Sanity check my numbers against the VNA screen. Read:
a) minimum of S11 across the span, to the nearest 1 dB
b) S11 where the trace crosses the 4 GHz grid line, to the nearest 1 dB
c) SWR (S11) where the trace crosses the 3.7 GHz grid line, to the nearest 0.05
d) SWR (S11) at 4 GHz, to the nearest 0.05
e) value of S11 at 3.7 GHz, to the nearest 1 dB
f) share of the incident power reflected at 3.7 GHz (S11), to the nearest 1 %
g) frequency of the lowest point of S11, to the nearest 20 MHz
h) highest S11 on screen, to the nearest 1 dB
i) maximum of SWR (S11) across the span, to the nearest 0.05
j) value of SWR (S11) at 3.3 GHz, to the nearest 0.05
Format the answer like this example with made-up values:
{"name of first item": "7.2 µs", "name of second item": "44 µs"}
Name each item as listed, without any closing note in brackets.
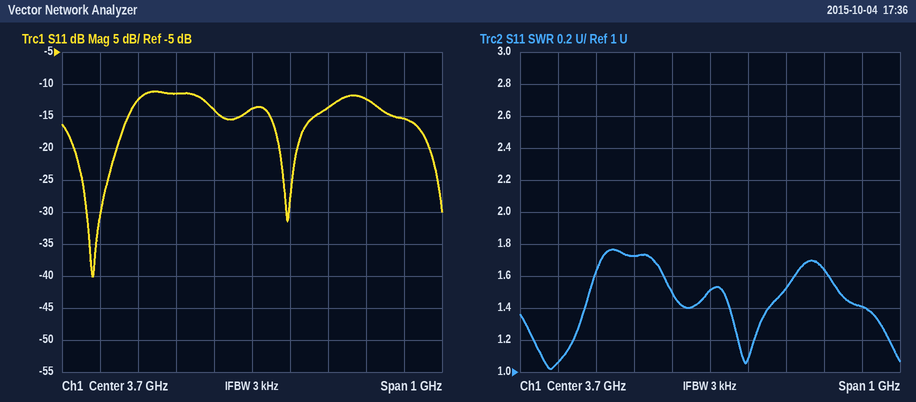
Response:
{"minimum of S11 across the span, to the nearest 1 dB": "-40 dB", "S11 where the trace crosses the 4 GHz grid line, to the nearest 1 dB": "-12 dB", "SWR (S11) where the trace crosses the 3.7 GHz grid line, to the nearest 0.05": "1.50", "SWR (S11) at 4 GHz, to the nearest 0.05": "1.65", "value of S11 at 3.7 GHz, to the nearest 1 dB": "-14 dB", "share of the incident power reflected at 3.7 GHz (S11), to the nearest 1 %": "4 %", "frequency of the lowest point of S11, to the nearest 20 MHz": "3.28 GHz", "highest S11 on screen, to the nearest 1 dB": "-11 dB", "maximum of SWR (S11) across the span, to the nearest 0.05": "1.75", "value of SWR (S11) at 3.3 GHz, to the nearest 0.05": "1.05"}
